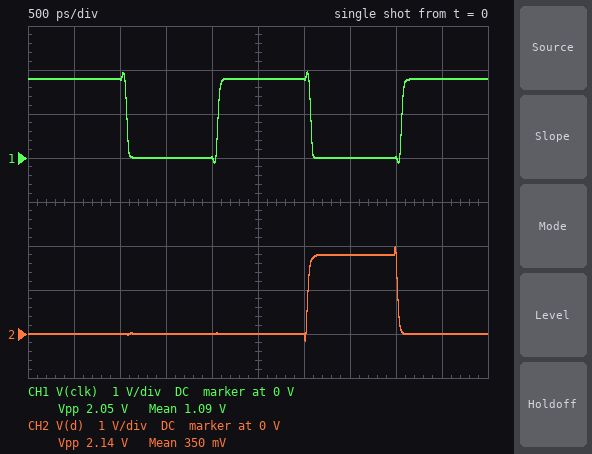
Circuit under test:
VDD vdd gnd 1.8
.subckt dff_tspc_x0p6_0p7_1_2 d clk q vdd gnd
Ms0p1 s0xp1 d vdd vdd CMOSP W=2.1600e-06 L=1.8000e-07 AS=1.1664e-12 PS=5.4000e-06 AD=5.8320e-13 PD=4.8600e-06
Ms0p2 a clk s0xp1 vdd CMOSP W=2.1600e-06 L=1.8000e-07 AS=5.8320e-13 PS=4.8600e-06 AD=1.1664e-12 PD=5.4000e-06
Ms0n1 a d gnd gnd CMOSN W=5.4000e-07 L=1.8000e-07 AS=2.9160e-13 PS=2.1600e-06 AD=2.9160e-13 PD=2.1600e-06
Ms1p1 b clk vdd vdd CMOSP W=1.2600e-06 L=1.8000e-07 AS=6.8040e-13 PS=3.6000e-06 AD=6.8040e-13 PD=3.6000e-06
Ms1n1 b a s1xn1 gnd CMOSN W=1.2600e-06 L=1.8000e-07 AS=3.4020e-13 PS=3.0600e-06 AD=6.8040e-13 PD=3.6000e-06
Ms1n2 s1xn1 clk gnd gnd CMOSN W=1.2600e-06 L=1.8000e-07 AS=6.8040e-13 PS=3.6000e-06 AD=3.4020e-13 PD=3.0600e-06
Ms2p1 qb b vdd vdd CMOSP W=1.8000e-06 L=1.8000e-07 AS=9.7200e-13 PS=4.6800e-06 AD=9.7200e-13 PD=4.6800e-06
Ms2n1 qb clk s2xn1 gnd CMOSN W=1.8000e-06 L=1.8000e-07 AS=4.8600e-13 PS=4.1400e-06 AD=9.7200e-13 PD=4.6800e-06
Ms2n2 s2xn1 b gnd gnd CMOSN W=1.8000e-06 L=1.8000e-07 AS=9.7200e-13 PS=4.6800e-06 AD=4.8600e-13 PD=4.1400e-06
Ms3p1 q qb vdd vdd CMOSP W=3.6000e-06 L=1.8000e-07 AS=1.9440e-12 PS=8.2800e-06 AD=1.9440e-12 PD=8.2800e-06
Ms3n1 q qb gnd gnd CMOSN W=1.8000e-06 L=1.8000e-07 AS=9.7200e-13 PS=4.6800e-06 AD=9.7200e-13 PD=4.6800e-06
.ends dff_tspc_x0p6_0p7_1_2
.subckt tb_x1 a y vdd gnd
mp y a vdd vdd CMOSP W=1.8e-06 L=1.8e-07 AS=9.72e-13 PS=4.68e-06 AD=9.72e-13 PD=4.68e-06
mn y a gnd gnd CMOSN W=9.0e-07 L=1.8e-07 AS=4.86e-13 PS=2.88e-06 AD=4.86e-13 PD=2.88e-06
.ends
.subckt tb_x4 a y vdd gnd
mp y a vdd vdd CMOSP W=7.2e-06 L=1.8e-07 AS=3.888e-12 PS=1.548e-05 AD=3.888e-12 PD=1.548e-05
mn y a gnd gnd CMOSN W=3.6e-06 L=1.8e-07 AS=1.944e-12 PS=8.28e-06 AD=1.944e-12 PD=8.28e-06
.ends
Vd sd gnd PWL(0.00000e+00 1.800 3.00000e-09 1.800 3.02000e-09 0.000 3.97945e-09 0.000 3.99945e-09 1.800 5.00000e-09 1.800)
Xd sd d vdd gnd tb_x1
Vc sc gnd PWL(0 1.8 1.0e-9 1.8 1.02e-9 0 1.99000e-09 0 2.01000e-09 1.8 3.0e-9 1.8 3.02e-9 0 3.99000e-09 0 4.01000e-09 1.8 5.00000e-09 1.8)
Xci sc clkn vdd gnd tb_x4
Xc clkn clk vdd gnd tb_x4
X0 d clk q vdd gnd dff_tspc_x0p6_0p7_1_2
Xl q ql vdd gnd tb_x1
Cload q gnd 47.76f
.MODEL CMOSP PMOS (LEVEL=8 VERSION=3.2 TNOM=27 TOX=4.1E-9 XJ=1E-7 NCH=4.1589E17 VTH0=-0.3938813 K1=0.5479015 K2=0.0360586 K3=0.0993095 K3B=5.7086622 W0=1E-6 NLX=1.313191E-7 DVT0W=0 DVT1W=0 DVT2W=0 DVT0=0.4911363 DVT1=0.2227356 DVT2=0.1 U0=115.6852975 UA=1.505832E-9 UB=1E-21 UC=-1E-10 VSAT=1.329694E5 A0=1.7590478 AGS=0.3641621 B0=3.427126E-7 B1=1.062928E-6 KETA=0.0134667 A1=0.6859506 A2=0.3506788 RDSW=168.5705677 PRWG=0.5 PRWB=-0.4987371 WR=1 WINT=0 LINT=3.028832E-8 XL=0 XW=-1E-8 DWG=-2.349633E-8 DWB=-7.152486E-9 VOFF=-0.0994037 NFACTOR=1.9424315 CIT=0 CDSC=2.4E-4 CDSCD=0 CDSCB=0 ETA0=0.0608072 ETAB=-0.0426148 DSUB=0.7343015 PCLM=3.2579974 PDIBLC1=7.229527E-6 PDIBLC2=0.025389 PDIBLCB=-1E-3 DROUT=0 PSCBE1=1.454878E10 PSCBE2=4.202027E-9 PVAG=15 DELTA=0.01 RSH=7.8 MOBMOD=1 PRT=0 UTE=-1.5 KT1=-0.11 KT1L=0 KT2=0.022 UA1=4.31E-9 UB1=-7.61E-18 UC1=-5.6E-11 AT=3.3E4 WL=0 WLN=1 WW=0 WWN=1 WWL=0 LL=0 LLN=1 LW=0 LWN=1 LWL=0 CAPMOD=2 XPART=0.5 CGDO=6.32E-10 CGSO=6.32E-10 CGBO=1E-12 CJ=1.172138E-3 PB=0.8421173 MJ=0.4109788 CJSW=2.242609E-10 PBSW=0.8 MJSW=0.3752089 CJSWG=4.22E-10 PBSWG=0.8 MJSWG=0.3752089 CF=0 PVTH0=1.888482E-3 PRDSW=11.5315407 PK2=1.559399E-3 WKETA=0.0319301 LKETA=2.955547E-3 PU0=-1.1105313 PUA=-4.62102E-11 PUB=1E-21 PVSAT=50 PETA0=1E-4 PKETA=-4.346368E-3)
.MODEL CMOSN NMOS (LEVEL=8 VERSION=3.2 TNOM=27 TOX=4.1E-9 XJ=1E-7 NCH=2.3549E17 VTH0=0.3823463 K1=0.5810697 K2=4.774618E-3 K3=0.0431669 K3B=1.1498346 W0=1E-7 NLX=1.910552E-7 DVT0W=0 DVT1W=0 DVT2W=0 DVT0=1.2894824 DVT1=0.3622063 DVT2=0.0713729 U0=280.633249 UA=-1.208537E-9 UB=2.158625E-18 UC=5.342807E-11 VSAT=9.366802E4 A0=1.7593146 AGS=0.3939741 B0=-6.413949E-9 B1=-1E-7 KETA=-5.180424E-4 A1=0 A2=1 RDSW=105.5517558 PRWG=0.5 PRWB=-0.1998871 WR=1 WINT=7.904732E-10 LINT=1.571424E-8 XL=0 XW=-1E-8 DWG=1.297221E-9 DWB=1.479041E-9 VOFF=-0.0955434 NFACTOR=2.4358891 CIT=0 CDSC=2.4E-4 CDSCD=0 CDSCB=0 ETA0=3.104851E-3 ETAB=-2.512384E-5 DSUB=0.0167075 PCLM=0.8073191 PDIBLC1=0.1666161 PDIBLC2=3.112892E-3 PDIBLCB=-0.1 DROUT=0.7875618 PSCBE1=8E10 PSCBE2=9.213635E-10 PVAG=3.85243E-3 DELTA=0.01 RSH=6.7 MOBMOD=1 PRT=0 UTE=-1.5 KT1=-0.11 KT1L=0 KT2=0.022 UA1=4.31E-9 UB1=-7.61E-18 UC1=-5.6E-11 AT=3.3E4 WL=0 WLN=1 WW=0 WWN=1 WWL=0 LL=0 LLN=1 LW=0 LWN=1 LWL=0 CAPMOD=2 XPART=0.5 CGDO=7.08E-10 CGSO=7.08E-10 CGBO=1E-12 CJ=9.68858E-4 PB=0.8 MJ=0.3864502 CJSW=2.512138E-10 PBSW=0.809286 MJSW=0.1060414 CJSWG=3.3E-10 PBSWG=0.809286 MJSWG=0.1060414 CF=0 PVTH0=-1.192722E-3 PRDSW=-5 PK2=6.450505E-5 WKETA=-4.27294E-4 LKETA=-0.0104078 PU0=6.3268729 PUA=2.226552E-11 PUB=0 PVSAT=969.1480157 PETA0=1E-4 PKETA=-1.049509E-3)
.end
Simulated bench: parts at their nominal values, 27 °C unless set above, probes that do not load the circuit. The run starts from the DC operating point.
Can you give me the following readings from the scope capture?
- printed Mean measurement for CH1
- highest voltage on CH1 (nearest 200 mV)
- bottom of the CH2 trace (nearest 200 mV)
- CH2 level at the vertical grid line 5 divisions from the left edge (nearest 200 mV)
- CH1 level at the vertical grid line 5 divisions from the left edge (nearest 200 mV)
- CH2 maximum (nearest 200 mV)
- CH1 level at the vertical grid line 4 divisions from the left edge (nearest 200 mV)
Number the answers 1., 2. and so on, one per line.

1. 1.09 V
2. 2.0 V
3. -200 mV
4. 0 V
5. 1.8 V
6. 2.0 V
7. 0 V
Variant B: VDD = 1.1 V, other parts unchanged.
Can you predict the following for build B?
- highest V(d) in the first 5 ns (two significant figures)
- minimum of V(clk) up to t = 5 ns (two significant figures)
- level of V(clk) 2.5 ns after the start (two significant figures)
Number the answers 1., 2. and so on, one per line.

1. 1.3 V
2. -210 mV
3. 1.1 V
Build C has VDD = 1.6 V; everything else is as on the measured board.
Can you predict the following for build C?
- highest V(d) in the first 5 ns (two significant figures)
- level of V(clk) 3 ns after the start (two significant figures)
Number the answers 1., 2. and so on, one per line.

1. 1.8 V
2. 1.6 V
